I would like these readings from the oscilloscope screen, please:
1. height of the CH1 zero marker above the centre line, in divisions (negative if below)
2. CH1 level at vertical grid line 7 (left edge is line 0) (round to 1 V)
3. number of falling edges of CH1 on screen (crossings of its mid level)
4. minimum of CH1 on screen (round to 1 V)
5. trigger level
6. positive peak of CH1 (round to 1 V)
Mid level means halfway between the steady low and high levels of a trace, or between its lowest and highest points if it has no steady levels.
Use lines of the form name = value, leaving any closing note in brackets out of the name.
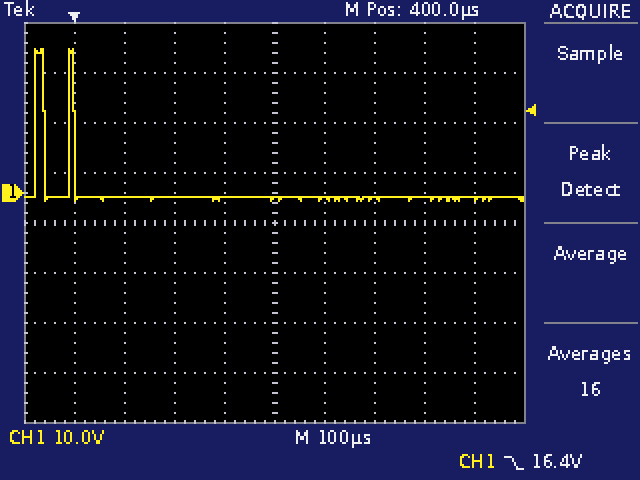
height of the CH1 zero marker above the centre line, in divisions = +0.6 div
CH1 level at vertical grid line 7 (left edge is line 0) = -1 V
number of falling edges of CH1 on screen = 2
minimum of CH1 on screen = -2 V
trigger level = 16.4 V
positive peak of CH1 = 29 V
